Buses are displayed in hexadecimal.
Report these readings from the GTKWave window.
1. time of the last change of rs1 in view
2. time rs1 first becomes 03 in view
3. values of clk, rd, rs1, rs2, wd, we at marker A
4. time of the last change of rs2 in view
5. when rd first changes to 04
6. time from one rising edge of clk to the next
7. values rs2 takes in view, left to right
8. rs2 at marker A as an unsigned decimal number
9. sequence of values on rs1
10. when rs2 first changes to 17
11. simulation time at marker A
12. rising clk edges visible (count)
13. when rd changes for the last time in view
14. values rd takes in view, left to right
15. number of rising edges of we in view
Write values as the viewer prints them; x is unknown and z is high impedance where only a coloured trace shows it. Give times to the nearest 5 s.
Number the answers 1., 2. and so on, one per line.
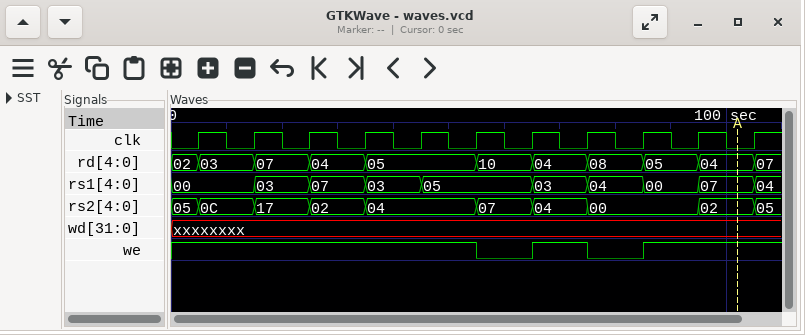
1. 105 s
2. 15 s
3. clk=0, rd=04, rs1=07, rs2=02, wd=xxxxxxxx, we=1
4. 105 s
5. 25 s
6. 10 s
7. 05, 0C, 17, 02, 04, 07, 04, 00, 02, 05
8. 2
9. 00, 03, 07, 03, 05, 03, 04, 00, 07, 04
10. 15 s
11. 100 s
12. 11
13. 105 s
14. 02, 03, 07, 04, 05, 10, 04, 08, 05, 04, 07
15. 2
